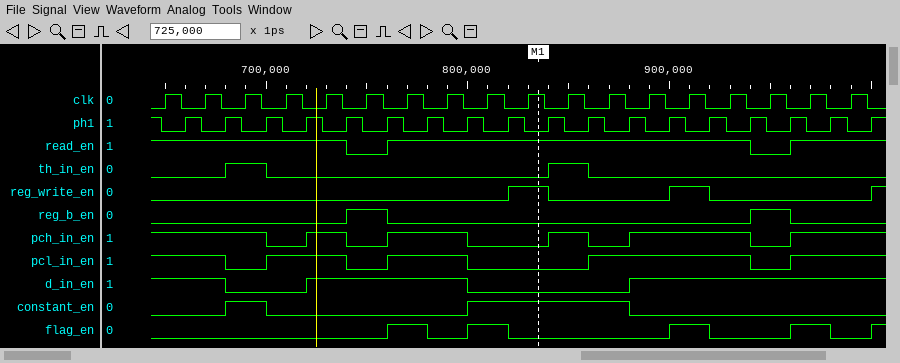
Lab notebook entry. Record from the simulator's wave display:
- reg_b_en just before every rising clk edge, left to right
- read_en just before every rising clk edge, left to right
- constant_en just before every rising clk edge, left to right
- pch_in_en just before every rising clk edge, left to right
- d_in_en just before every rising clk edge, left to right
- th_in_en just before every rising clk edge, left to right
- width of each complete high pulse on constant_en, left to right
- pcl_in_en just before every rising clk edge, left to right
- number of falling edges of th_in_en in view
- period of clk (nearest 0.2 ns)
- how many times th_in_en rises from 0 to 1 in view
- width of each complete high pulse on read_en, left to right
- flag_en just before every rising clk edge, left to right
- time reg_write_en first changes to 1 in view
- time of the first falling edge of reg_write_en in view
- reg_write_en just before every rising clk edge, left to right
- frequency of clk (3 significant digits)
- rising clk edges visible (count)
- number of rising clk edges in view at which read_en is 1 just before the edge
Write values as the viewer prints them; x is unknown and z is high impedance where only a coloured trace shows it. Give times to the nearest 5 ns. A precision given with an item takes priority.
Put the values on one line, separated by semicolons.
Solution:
0 0 0 0 0 1 0 0 0 0 0 0 0 0 0 1 0 0; 1 1 1 1 1 0 1 1 1 1 1 1 1 1 1 0 1 1; 0 0 1 0 0 0 0 0 1 1 1 1 0 0 0 0 0 0; 1 1 1 0 1 0 1 1 0 0 1 0 1 1 1 0 1 1; 1 1 0 0 1 1 1 1 0 0 0 0 1 1 1 1 1 1; 0 0 1 0 0 0 0 0 0 0 1 0 0 0 0 0 0 0; 20 ns, 80 ns; 1 1 0 1 1 0 1 1 0 0 0 1 1 1 1 0 1 1; 2; 20 ns; 2; 180 ns; 0 0 0 0 0 0 1 0 1 0 0 0 0 1 0 0 1 0; 820 ns; 840 ns; 0 0 0 0 0 0 0 0 0 1 0 0 0 1 0 0 0 0; 50.0 MHz; 18; 16
